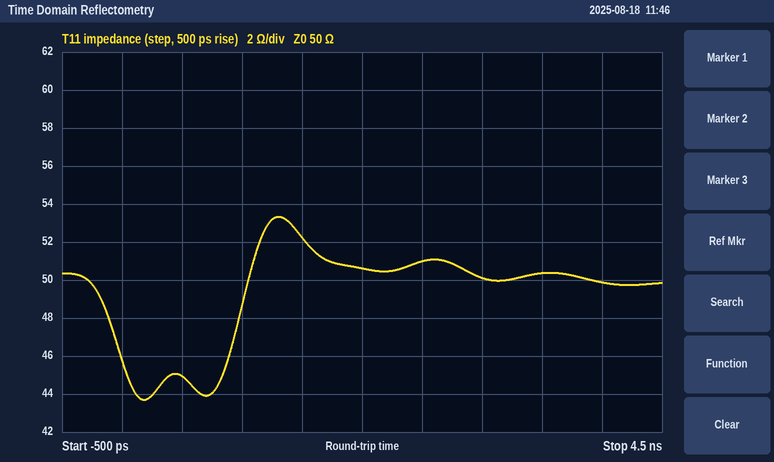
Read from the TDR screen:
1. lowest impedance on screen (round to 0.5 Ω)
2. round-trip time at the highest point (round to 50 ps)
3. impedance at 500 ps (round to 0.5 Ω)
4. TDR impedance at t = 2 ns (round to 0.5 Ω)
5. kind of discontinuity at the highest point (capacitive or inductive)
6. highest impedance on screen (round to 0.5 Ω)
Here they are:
43.5 Ω
1.30 ns
45.0 Ω
50.5 Ω
inductive
53.5 Ω
